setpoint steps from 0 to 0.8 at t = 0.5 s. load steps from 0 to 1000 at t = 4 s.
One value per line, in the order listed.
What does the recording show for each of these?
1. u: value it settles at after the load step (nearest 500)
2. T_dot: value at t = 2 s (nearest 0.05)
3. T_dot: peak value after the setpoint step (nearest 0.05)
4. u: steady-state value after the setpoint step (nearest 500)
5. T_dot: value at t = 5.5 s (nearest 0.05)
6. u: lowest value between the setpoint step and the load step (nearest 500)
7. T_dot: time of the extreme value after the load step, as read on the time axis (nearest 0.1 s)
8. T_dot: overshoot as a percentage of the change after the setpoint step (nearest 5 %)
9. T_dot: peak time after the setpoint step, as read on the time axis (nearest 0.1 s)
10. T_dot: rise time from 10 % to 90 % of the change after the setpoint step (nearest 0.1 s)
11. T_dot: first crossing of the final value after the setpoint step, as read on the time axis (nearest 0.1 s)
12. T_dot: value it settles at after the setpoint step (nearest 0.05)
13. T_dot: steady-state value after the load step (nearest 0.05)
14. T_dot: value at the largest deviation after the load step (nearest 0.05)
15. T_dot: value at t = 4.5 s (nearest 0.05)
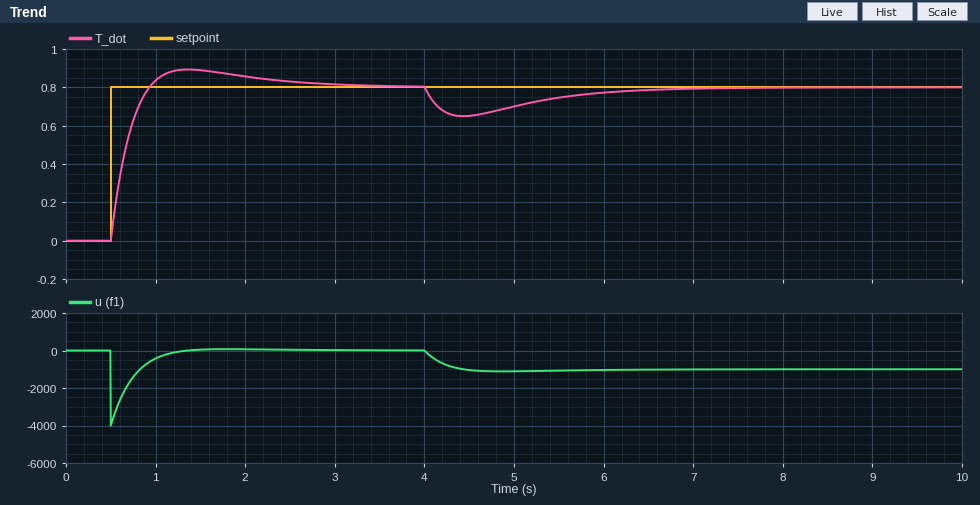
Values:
-1000
0.85
0.90
0
0.75
-4000
4.4 s
10 %
1.4 s
0.3 s
0.9 s
0.80
0.80
0.65
0.65
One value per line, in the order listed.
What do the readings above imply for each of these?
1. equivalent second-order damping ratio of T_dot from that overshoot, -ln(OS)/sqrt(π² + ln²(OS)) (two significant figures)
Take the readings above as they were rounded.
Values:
0.59
